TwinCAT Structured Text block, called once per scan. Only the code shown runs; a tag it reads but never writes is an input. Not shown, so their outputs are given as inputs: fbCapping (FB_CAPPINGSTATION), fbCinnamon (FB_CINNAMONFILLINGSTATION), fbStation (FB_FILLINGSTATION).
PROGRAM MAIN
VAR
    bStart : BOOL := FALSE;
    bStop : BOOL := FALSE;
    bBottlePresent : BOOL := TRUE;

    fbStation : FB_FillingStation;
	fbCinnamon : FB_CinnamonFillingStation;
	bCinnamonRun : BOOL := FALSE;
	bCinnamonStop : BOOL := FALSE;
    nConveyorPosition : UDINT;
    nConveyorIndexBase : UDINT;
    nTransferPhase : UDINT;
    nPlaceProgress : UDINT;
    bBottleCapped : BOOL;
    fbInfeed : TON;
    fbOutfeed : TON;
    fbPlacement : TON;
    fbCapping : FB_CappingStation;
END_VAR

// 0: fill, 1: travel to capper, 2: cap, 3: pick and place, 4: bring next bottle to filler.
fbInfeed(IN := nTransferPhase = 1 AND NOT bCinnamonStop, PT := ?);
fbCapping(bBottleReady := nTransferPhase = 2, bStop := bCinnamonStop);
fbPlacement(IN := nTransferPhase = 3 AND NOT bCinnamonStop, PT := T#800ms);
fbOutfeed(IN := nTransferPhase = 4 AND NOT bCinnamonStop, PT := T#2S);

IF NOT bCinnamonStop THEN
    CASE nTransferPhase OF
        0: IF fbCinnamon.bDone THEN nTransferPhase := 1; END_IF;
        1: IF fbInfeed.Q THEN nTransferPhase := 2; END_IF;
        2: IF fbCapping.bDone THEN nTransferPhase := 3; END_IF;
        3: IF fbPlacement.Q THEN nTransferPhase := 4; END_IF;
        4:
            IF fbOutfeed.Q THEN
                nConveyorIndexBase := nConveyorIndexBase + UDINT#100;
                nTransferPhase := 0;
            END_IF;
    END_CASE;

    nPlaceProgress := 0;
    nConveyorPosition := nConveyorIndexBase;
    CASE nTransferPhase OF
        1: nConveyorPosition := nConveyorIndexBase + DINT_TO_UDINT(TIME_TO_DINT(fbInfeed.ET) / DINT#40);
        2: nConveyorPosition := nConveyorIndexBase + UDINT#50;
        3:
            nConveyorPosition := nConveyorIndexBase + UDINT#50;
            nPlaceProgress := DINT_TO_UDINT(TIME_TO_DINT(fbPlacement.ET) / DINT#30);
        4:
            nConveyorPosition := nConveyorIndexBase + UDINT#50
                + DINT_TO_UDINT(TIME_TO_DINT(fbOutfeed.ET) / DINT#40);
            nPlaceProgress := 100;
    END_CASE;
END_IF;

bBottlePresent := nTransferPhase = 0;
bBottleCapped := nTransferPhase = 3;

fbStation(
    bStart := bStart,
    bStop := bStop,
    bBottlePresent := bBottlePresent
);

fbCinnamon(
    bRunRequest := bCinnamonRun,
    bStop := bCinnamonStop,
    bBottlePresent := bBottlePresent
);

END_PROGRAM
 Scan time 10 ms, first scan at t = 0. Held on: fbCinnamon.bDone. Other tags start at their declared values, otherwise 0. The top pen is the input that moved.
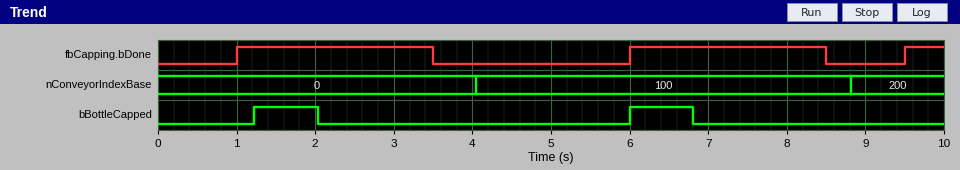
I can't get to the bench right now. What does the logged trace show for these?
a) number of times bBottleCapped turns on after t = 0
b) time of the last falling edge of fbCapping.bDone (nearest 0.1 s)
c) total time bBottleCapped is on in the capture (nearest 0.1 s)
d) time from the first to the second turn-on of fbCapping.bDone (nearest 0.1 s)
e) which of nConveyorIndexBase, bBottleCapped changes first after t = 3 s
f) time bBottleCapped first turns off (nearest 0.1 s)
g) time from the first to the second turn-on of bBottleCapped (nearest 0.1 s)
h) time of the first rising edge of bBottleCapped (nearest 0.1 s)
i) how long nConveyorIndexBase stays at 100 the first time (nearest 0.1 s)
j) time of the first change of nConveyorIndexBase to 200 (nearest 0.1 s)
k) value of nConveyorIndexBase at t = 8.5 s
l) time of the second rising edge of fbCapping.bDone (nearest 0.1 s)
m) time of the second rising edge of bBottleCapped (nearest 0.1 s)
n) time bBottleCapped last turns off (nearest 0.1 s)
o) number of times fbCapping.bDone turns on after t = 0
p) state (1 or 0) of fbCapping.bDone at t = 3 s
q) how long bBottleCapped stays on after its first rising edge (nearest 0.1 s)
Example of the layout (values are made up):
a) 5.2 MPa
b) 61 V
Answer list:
a) 2
b) 8.5 s
c) 1.6 s
d) 5.0 s
e) nConveyorIndexBase
f) 2.0 s
g) 4.8 s
h) 1.2 s
i) 4.8 s
j) 8.8 s
k) 100
l) 6.0 s
m) 6.0 s
n) 6.8 s
o) 3
p) 1
q) 0.8 s
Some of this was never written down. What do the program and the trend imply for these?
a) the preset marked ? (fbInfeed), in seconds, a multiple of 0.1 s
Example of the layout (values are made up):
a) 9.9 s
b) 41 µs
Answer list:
a) 1.2 s
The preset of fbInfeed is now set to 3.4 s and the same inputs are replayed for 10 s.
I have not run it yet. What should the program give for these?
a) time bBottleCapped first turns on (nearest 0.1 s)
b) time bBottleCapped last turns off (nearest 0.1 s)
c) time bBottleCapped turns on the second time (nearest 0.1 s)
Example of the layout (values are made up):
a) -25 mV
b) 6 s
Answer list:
a) 3.4 s
b) 4.2 s
c) 9.7 s
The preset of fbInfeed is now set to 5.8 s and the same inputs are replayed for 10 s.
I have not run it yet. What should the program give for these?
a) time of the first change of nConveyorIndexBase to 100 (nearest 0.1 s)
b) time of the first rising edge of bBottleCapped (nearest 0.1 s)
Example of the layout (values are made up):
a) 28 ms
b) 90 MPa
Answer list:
a) 8.8 s
b) 6.0 s
